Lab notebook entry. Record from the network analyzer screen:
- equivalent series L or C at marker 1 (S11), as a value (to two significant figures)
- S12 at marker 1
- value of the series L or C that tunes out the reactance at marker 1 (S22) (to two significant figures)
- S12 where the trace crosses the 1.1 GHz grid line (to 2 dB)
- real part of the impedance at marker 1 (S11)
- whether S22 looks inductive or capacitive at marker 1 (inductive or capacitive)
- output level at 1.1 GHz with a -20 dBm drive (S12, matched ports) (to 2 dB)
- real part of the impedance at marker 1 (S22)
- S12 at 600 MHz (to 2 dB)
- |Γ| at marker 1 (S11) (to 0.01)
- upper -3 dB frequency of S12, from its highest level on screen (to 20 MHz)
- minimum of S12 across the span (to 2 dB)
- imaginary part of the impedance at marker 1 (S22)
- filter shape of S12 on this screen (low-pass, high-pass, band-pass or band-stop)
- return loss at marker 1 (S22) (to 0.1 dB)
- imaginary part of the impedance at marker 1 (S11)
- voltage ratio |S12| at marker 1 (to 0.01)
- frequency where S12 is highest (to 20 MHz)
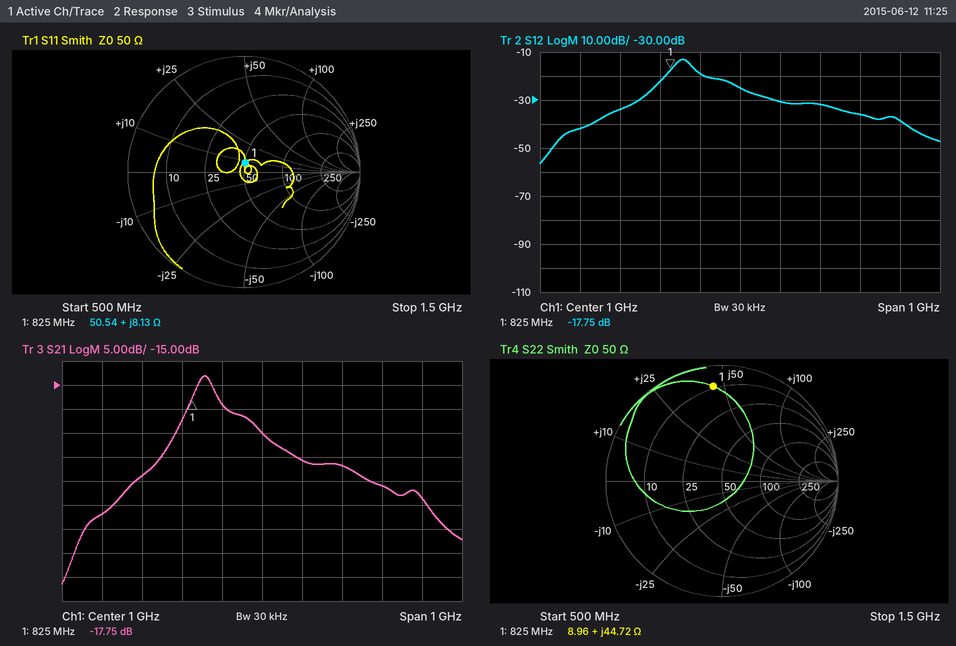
1.6 nH
-17.75 dB
4.3 pF
-30 dB
50.54 Ω
inductive
-50 dBm
8.96 Ω
-42 dB
0.08
880 MHz
-56 dB
+44.72 Ω
band-pass
1.7 dB
+8.13 Ω
0.13
860 MHz
